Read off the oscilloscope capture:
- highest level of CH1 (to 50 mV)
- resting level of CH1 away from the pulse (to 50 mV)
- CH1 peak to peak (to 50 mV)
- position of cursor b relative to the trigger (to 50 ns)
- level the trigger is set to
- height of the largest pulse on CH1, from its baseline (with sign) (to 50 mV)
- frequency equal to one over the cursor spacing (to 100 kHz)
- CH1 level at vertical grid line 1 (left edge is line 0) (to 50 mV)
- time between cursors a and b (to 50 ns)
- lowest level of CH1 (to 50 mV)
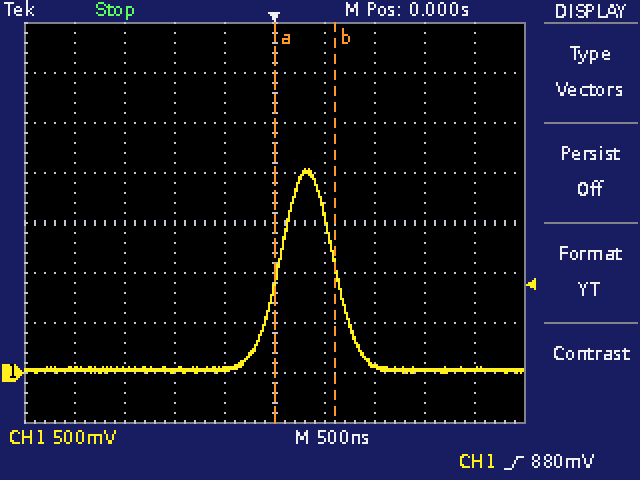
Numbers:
2.05 V
50 mV
2.05 V
+600 ns
880 mV
+2.00 V
1.7 MHz
50 mV
600 ns
0 mV
